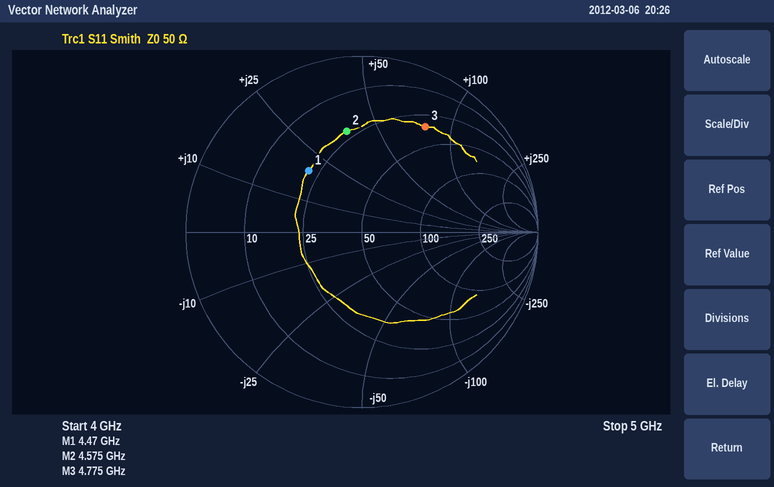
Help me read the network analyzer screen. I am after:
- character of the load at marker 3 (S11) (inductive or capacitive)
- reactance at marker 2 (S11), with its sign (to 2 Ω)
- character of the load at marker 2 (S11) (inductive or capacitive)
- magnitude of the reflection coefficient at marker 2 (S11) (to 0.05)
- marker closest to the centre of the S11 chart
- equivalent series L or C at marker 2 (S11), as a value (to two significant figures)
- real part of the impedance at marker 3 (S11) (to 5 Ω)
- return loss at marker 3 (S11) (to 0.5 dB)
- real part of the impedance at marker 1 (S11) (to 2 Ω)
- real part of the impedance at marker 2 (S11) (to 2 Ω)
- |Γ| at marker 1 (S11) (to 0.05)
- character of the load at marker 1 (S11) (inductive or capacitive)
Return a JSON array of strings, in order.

["inductive", "+38 Ω", "inductive", "0.60", "marker 1", "1.3 nH", "35 Ω", "3.0 dB", "22 Ω", "22 Ω", "0.45", "inductive"]
